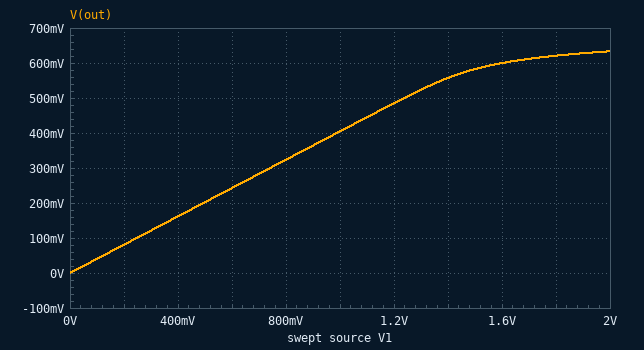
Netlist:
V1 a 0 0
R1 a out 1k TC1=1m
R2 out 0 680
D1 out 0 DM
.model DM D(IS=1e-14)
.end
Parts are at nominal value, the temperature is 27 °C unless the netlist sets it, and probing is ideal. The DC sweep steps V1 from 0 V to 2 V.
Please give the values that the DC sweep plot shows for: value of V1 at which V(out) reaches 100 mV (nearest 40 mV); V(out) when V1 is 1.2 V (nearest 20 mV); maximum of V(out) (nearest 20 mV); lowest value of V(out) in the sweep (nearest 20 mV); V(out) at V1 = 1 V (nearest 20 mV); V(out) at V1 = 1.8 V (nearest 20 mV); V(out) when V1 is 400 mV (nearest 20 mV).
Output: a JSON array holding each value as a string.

["240 mV", "480 mV", "640 mV", "0 V", "400 mV", "620 mV", "160 mV"]
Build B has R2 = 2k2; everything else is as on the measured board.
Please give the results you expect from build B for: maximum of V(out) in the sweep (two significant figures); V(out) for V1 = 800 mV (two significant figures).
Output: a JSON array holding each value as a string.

["660 mV", "540 mV"]
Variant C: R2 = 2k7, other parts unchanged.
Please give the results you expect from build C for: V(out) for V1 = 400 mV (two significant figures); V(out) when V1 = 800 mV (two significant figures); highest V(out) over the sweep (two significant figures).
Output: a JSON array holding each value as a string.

["290 mV", "560 mV", "660 mV"]
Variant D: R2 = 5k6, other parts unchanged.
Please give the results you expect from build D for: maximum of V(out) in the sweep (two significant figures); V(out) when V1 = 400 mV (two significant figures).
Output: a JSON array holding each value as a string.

["660 mV", "340 mV"]
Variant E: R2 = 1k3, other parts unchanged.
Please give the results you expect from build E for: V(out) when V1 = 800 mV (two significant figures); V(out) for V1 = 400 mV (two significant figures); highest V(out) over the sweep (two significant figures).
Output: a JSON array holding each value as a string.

["450 mV", "230 mV", "650 mV"]
